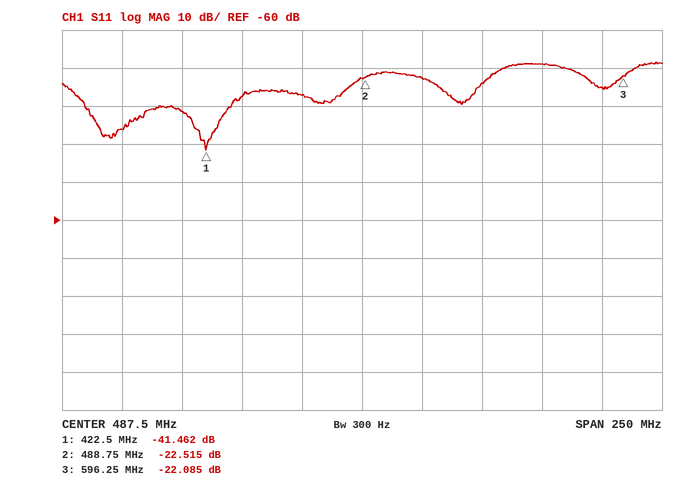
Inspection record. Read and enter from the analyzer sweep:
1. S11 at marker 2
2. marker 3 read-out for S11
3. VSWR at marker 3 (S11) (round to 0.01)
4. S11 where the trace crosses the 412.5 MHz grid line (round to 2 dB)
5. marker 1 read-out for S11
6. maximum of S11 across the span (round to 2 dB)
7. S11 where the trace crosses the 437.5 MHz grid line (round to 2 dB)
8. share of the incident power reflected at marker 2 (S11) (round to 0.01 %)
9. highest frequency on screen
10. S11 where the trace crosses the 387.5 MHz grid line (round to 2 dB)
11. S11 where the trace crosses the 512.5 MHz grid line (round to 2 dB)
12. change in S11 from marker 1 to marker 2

-22.515 dB
-22.085 dB
1.17
-32 dB
-41.462 dB
-18 dB
-28 dB
0.56 %
612.5 MHz
-36 dB
-22 dB
18.947 dB
